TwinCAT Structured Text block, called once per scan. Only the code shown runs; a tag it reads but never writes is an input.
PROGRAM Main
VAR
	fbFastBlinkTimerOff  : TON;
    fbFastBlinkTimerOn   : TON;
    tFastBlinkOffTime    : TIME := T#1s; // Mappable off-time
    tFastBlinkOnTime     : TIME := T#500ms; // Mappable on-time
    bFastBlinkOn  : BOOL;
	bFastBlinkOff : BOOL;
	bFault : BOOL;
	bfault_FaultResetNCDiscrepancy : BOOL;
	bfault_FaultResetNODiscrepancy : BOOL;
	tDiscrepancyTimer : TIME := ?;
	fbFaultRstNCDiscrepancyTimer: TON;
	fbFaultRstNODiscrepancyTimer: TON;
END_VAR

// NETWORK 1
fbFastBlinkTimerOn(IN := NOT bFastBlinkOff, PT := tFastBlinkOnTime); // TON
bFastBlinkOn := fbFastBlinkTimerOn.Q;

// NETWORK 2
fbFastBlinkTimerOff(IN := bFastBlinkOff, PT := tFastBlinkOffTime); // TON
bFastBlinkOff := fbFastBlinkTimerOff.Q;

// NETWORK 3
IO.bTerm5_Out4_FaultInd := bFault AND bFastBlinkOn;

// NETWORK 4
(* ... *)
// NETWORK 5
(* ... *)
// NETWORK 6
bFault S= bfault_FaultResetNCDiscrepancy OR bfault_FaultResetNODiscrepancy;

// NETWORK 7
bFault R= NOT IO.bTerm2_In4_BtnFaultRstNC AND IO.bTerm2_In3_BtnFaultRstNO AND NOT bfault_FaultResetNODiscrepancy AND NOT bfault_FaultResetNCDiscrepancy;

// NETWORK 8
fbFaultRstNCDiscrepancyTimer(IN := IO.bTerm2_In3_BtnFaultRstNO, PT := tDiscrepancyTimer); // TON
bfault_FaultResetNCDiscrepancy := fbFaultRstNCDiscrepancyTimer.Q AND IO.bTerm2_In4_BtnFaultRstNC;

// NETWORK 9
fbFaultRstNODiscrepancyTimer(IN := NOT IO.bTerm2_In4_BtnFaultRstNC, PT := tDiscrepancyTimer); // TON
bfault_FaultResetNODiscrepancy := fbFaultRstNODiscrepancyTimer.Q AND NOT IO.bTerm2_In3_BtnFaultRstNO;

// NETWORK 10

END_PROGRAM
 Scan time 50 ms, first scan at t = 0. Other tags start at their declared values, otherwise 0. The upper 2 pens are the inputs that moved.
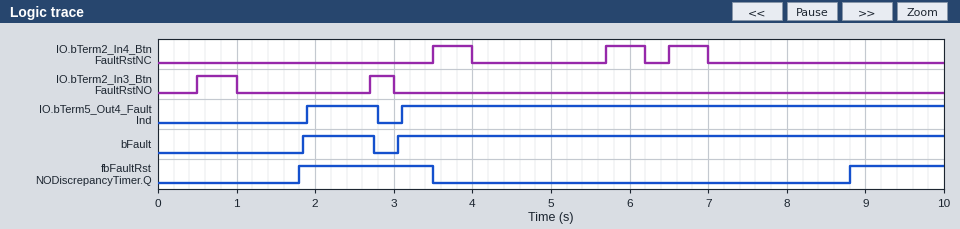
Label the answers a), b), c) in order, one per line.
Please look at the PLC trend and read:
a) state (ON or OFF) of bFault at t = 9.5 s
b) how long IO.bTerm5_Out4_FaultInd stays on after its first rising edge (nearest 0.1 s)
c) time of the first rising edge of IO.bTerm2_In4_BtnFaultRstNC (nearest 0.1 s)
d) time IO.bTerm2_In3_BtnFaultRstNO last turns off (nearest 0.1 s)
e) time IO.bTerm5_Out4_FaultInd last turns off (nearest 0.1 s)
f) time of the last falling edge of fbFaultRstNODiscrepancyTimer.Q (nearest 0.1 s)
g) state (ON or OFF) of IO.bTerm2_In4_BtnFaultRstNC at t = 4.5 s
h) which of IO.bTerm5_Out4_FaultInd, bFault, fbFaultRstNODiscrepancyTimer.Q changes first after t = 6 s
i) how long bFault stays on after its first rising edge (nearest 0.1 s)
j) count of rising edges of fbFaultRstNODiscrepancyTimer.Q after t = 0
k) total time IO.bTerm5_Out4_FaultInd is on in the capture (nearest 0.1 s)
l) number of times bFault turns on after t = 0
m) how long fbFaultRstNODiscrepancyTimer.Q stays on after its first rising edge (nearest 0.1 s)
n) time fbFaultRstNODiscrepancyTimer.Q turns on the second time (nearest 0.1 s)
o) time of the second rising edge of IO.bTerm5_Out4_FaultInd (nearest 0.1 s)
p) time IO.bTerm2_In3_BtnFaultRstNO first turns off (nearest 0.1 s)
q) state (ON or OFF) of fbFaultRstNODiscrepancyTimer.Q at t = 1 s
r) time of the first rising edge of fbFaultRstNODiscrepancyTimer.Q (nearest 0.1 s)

a) ON
b) 0.9 s
c) 3.5 s
d) 3.0 s
e) 2.8 s
f) 3.5 s
g) OFF
h) fbFaultRstNODiscrepancyTimer.Q
i) 0.9 s
j) 2
k) 7.8 s
l) 2
m) 1.7 s
n) 8.8 s
o) 3.1 s
p) 1.0 s
q) OFF
r) 1.8 s
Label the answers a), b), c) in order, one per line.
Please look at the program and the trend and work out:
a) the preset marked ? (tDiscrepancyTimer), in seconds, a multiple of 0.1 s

a) 1.8 s
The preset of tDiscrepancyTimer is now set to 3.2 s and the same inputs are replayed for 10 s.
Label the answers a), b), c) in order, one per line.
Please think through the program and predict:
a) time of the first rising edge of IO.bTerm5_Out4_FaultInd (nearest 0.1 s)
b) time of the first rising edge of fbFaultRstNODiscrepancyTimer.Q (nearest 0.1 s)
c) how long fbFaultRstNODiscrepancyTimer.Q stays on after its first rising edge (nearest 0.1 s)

a) 3.3 s
b) 3.2 s
c) 0.3 s
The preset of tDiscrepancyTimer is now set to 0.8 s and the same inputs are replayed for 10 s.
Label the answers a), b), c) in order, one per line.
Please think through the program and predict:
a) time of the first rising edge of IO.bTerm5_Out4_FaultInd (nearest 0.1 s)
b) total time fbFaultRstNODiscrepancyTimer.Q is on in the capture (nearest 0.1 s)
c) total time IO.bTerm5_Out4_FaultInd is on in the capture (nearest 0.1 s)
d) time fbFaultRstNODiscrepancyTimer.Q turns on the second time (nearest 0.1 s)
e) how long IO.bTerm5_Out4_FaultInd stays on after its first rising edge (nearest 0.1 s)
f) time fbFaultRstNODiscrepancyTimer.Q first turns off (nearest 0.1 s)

a) 1.1 s
b) 5.8 s
c) 8.6 s
d) 4.8 s
e) 1.7 s
f) 3.5 s
